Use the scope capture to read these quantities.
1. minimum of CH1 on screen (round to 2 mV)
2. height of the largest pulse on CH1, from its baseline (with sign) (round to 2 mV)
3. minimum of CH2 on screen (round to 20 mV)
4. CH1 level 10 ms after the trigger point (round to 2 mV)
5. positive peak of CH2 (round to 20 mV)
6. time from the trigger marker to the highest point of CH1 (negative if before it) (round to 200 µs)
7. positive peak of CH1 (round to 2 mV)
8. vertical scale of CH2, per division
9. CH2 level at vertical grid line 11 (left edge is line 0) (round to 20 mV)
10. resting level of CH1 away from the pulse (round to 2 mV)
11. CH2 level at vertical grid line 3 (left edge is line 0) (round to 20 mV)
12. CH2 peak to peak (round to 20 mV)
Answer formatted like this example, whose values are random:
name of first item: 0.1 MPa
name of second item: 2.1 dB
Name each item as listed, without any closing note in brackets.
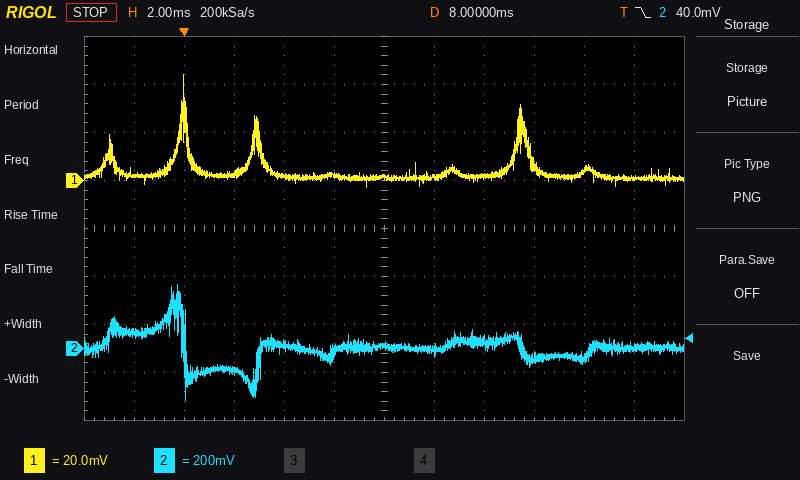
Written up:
minimum of CH1 on screen: -2 mV
height of the largest pulse on CH1, from its baseline (with sign): +42 mV
minimum of CH2 on screen: -220 mV
CH1 level 10 ms after the trigger point: 2 mV
positive peak of CH2: 260 mV
time from the trigger marker to the highest point of CH1 (negative if before it): 0.0 ms
positive peak of CH1: 44 mV
vertical scale of CH2, per division: 200 mV
CH2 level at vertical grid line 11 (left edge is line 0): 0 mV
resting level of CH1 away from the pulse: 2 mV
CH2 level at vertical grid line 3 (left edge is line 0): -100 mV
CH2 peak to peak: 480 mV
